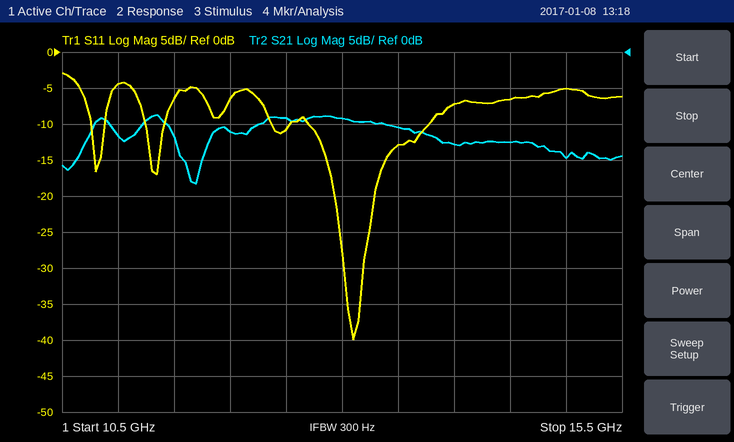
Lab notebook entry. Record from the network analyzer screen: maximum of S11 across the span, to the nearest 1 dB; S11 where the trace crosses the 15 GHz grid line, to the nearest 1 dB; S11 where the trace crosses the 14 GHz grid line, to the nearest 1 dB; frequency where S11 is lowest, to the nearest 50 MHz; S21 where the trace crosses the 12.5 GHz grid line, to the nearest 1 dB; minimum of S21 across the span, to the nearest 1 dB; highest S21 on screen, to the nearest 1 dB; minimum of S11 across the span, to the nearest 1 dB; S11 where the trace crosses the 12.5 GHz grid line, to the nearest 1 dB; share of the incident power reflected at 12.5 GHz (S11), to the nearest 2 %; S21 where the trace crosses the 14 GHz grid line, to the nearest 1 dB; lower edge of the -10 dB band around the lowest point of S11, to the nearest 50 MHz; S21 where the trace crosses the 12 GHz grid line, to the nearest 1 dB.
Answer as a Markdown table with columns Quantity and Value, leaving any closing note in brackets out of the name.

| Quantity | Value |
|---|---|
| maximum of S11 across the span, to the nearest 1 dB | -3 dB |
| S11 where the trace crosses the 15 GHz grid line, to the nearest 1 dB | -5 dB |
| S11 where the trace crosses the 14 GHz grid line, to the nearest 1 dB | -7 dB |
| frequency where S11 is lowest, to the nearest 50 MHz | 13.10 GHz |
| S21 where the trace crosses the 12.5 GHz grid line, to the nearest 1 dB | -9 dB |
| minimum of S21 across the span, to the nearest 1 dB | -18 dB |
| highest S21 on screen, to the nearest 1 dB | -9 dB |
| minimum of S11 across the span, to the nearest 1 dB | -40 dB |
| S11 where the trace crosses the 12.5 GHz grid line, to the nearest 1 dB | -11 dB |
| share of the incident power reflected at 12.5 GHz (S11), to the nearest 2 % | 8 % |
| S21 where the trace crosses the 14 GHz grid line, to the nearest 1 dB | -13 dB |
| lower edge of the -10 dB band around the lowest point of S11, to the nearest 50 MHz | 12.70 GHz |
| S21 where the trace crosses the 12 GHz grid line, to the nearest 1 dB | -11 dB |
